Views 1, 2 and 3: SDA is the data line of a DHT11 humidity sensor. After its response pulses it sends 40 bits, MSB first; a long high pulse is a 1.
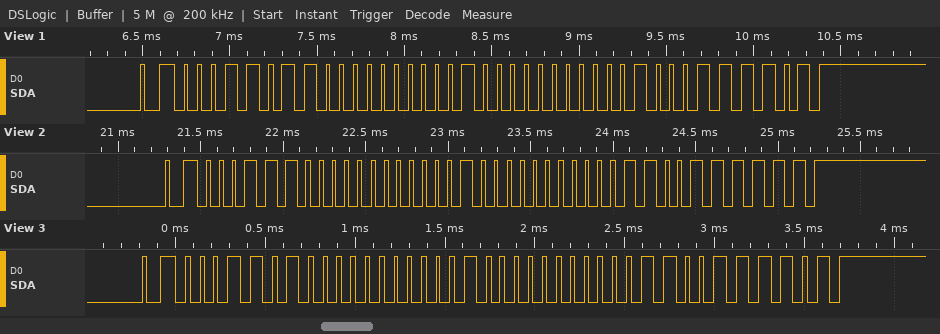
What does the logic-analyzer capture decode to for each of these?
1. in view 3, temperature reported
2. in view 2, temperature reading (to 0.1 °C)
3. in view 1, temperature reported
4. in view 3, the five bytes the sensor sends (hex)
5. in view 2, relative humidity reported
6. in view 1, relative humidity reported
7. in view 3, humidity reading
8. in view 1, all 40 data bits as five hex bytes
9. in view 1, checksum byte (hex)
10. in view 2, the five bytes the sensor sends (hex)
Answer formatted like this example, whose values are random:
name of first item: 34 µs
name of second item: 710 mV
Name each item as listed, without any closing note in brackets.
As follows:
in view 3, temperature reported: 32.3 °C
in view 2, temperature reading: 32.3 °C
in view 1, temperature reported: 32.2 °C
in view 3, the five bytes the sensor sends: 1A 00 20 03 3D
in view 2, relative humidity reported: 28 %
in view 1, relative humidity reported: 27 %
in view 3, humidity reading: 26 %
in view 1, all 40 data bits as five hex bytes: 1B 00 20 02 3D
in view 1, checksum byte: 0x3D
in view 2, the five bytes the sensor sends: 1C 00 20 03 3F
